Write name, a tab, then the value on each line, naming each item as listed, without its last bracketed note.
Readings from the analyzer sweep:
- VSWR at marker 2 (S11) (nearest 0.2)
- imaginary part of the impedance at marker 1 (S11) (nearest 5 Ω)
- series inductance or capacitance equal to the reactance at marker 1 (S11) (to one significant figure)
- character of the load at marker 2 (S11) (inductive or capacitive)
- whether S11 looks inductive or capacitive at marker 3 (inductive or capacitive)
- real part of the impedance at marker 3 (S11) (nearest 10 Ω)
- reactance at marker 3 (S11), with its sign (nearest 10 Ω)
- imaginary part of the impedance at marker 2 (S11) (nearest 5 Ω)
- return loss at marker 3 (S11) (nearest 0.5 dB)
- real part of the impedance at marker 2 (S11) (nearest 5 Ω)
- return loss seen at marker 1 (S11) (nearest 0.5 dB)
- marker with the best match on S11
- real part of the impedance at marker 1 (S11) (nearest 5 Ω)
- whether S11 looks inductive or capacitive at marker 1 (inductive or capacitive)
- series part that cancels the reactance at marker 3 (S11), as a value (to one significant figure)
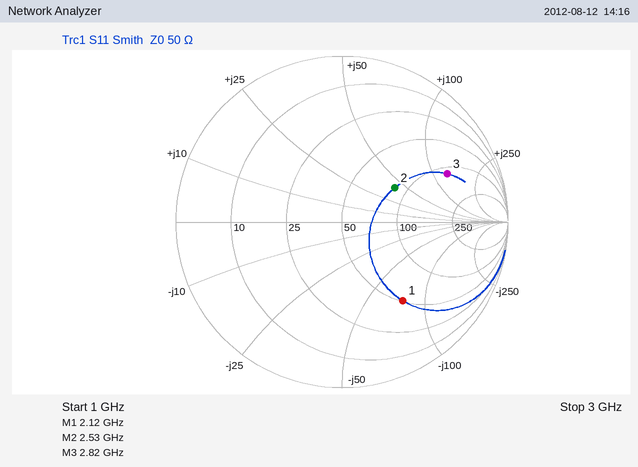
VSWR at marker 2 (S11)	2.2
imaginary part of the impedance at marker 1 (S11)	-75 Ω
series inductance or capacitance equal to the reactance at marker 1 (S11)	1.0 pF
character of the load at marker 2 (S11)	inductive
whether S11 looks inductive or capacitive at marker 3	inductive
real part of the impedance at marker 3 (S11)	120 Ω
reactance at marker 3 (S11), with its sign	+130 Ω
imaginary part of the impedance at marker 2 (S11)	+40 Ω
return loss at marker 3 (S11)	3.0 dB
real part of the impedance at marker 2 (S11)	85 Ω
return loss seen at marker 1 (S11)	4.5 dB
marker with the best match on S11	marker 2
real part of the impedance at marker 1 (S11)	50 Ω
whether S11 looks inductive or capacitive at marker 1	capacitive
series part that cancels the reactance at marker 3 (S11), as a value	400 fF
